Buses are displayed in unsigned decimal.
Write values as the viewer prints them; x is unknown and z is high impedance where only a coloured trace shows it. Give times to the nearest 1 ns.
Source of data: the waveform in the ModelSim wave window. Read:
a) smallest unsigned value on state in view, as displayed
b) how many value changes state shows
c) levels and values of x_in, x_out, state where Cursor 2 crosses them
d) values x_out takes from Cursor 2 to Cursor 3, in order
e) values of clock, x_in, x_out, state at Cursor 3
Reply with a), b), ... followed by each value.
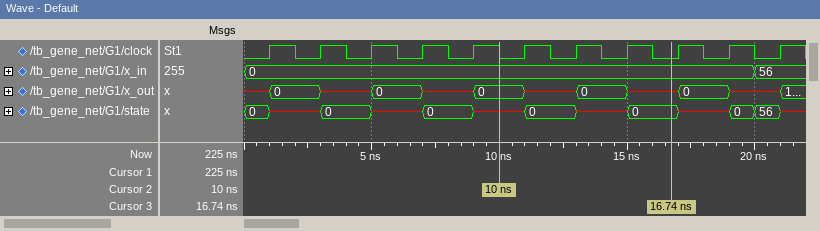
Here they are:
a) 0
b) 12
c) x_in=0, x_out=0, state=x
d) 0, x, 0, x
e) clock=0, x_in=0, x_out=x, state=0
